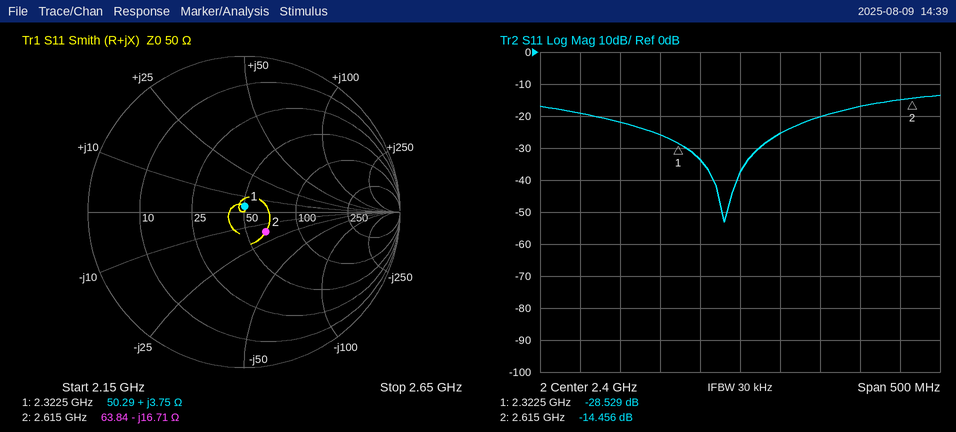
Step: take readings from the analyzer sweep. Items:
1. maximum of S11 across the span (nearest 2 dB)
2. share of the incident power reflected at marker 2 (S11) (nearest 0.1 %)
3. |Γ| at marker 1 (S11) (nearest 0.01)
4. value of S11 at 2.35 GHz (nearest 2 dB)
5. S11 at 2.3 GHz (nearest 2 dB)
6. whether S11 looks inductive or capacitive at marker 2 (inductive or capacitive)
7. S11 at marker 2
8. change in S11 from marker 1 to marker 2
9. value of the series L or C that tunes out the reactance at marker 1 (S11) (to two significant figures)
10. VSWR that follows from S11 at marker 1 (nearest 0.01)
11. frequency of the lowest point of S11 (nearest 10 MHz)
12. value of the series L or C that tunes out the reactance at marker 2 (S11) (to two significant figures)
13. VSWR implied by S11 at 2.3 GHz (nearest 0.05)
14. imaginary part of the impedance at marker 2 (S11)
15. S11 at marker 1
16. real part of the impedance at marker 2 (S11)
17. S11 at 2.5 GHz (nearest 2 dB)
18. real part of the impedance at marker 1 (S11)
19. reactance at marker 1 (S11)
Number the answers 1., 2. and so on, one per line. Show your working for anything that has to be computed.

1. -14 dB
2. 10^(-14.456/10) ≈ 3.6 %
3. 0.04
4. -34 dB
5. -26 dB
6. capacitive
7. -14.456 dB
8. -14.456 − (-28.529) = 14.073 dB
9. C = 1/(2π × 2.3225 GHz × 3.75 Ω) ≈ 18 pF
10. (1 + 0.0375)/(1 − 0.0375) ≈ 1.08
11. 2.38 GHz
12. L = 16.71 Ω/(2π × 2.615 GHz) ≈ 1.0 nH
13. |Γ| = 10^(-26/20) = 0.0501; VSWR = (1 + 0.0501)/(1 − 0.0501) ≈ 1.11, so 1.10 to the nearest 0.05
14. -16.71 Ω
15. -28.529 dB
16. 63.84 Ω
17. -20 dB
18. 50.29 Ω
19. +3.75 Ω
